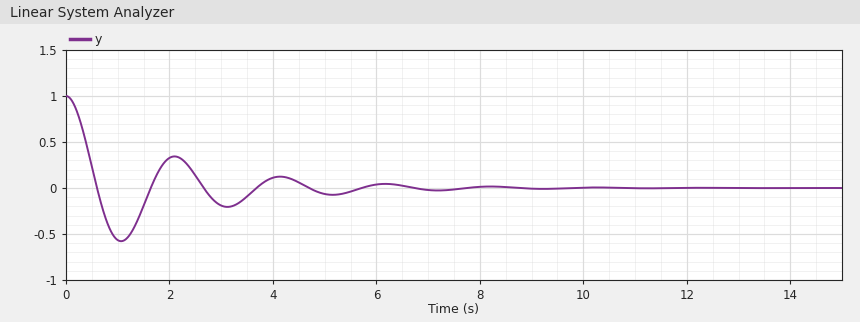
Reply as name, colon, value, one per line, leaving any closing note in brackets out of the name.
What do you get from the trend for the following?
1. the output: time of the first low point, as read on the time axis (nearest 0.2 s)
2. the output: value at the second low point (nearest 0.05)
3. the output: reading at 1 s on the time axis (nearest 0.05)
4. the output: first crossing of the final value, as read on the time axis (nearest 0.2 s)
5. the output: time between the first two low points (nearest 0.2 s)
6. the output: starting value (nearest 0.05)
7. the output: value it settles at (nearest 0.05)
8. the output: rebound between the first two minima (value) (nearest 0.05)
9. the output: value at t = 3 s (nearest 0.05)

the output: time of the first low point, as read on the time axis: 1.0 s
the output: value at the second low point: -0.20
the output: reading at 1 s on the time axis: -0.55
the output: first crossing of the final value, as read on the time axis: 0.6 s
the output: time between the first two low points: 2.0 s
the output: starting value: 1.00
the output: value it settles at: 0.00
the output: rebound between the first two minima (value): 0.35
the output: value at t = 3 s: -0.20
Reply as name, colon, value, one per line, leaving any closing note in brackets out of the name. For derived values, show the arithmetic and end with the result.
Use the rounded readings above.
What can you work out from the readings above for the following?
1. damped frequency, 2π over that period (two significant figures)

damped frequency, 2π over that period: 2π / 2 = 3.1 rad/s
